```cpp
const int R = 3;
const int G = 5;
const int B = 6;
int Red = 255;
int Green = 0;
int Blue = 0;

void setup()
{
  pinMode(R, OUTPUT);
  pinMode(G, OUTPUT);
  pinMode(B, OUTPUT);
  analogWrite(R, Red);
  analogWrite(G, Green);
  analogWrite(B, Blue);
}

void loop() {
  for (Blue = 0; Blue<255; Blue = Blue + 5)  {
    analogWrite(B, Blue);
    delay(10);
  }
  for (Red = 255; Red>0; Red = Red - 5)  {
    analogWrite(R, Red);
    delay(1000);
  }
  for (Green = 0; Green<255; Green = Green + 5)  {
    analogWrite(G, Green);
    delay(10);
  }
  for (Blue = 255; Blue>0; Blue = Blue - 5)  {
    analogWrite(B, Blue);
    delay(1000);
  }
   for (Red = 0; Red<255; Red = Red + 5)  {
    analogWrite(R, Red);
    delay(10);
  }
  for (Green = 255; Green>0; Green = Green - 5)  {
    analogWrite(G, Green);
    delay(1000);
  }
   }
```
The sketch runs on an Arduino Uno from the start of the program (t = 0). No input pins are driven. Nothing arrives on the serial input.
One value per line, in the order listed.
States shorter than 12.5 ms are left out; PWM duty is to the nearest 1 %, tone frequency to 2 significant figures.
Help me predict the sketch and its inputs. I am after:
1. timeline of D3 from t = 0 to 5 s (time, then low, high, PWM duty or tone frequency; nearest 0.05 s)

0 s high; 1.5 s PWM 98 %; 2.5 s PWM 96 %; 3.5 s PWM 94 %; 4.5 s PWM 92 %
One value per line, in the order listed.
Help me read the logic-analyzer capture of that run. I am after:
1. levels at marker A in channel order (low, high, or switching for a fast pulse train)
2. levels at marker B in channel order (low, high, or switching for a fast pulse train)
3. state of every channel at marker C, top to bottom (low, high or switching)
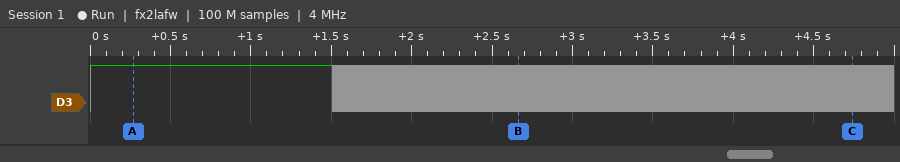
D3 high
D3 switching
D3 switching
